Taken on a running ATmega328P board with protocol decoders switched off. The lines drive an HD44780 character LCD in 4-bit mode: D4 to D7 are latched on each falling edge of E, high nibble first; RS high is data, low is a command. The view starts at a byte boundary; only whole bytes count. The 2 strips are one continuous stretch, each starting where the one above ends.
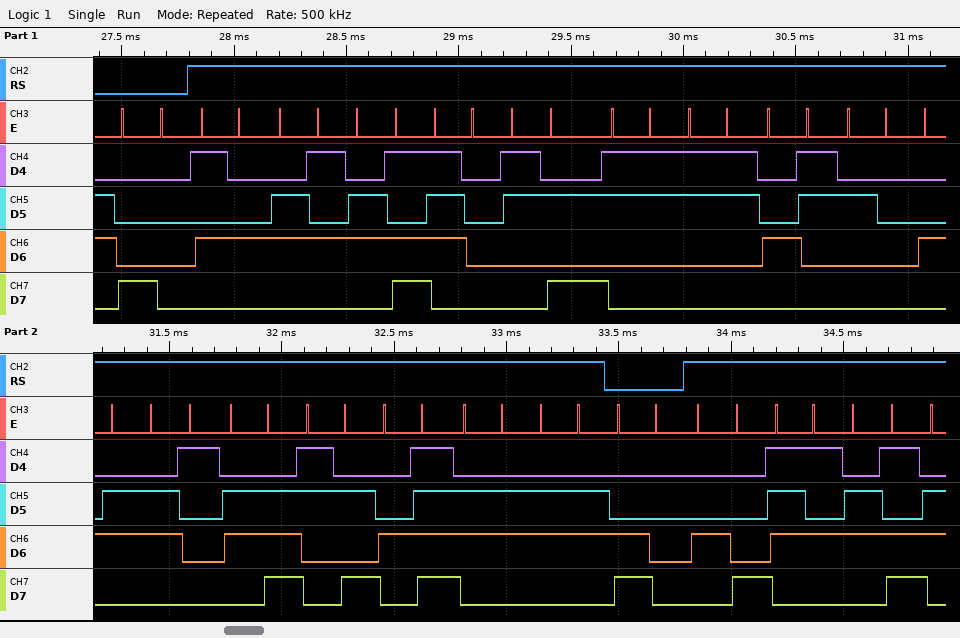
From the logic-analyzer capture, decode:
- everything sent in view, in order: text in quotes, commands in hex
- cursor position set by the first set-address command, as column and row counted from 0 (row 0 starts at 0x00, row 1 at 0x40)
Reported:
0x80 "Temp:33C Fan:Off" 0xC0 "Hum"
column 0, row 0
